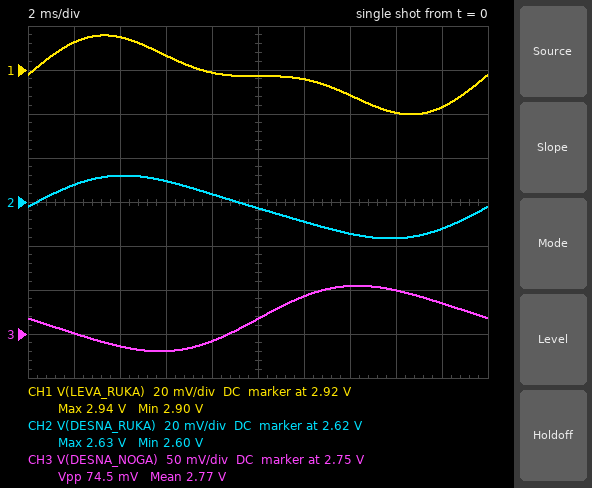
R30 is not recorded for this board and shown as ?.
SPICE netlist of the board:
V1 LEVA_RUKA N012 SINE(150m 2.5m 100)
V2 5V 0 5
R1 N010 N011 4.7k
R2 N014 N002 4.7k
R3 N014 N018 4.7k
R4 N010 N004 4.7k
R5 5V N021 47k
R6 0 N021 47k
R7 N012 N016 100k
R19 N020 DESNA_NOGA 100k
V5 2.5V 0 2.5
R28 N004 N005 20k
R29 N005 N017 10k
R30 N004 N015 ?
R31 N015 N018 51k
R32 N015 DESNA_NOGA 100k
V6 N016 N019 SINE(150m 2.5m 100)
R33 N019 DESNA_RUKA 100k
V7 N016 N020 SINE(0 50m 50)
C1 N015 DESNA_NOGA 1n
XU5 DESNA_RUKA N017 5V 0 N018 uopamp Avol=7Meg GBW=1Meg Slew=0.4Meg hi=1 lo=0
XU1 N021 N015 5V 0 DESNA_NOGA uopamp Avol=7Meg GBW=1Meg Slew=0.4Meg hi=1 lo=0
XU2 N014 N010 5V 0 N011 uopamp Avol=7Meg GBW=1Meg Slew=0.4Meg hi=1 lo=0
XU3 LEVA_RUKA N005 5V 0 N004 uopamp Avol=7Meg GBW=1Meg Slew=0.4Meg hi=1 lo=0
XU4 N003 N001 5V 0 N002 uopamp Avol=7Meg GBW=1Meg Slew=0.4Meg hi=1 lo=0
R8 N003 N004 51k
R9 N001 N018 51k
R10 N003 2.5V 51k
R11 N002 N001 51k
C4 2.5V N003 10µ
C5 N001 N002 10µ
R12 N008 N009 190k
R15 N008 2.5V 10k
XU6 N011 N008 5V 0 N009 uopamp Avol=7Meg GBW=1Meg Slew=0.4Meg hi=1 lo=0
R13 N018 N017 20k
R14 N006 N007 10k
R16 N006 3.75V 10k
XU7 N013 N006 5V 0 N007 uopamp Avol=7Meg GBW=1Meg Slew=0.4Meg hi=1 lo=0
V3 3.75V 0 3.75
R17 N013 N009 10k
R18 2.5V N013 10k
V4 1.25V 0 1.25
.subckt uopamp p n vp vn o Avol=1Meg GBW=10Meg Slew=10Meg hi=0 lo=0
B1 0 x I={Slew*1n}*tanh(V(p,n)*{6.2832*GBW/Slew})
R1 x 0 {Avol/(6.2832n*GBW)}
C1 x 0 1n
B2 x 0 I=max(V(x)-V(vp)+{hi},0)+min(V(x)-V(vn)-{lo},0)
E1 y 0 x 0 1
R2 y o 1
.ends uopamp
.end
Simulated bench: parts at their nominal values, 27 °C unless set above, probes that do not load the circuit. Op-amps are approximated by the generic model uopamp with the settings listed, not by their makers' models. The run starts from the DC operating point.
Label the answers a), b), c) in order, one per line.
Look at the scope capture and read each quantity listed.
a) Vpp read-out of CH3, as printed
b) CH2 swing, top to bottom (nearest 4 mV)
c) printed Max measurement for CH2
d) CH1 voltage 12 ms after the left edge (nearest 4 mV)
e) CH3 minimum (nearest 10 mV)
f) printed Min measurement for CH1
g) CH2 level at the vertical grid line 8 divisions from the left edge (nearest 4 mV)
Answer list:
a) 74.5 mV
b) 28 mV
c) 2.63 V
d) 2.916 V
e) 2.73 V
f) 2.90 V
g) 2.604 V
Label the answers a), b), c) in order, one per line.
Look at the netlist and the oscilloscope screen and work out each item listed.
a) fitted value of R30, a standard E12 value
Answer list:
a) 150 kΩ
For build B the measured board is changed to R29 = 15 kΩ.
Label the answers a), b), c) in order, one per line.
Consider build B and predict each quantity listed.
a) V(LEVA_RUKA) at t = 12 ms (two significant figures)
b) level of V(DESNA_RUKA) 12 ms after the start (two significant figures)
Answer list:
a) 2.8 V
b) 2.5 V
